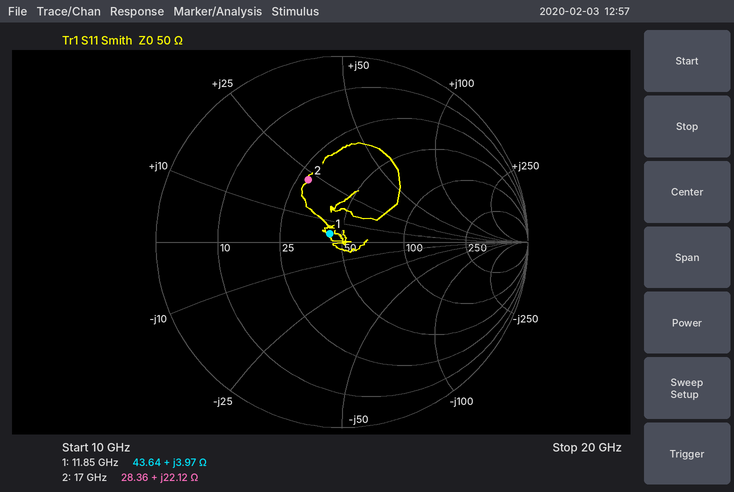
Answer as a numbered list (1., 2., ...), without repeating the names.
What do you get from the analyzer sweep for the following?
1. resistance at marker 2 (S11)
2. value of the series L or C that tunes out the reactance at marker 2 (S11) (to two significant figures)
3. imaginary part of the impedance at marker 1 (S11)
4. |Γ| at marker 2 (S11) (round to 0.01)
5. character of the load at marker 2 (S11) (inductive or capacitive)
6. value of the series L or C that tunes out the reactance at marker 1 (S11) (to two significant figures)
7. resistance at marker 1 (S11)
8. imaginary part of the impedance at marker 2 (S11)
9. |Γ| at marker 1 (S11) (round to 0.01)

1. 28.36 Ω
2. 420 fF
3. +3.97 Ω
4. 0.38
5. inductive
6. 3.4 pF
7. 43.64 Ω
8. +22.12 Ω
9. 0.08
